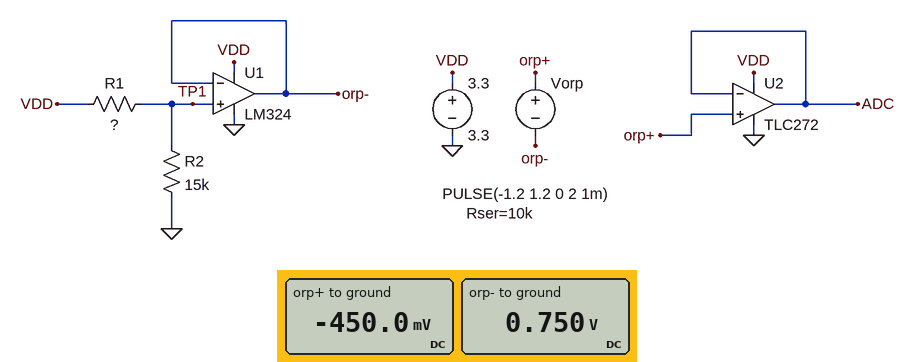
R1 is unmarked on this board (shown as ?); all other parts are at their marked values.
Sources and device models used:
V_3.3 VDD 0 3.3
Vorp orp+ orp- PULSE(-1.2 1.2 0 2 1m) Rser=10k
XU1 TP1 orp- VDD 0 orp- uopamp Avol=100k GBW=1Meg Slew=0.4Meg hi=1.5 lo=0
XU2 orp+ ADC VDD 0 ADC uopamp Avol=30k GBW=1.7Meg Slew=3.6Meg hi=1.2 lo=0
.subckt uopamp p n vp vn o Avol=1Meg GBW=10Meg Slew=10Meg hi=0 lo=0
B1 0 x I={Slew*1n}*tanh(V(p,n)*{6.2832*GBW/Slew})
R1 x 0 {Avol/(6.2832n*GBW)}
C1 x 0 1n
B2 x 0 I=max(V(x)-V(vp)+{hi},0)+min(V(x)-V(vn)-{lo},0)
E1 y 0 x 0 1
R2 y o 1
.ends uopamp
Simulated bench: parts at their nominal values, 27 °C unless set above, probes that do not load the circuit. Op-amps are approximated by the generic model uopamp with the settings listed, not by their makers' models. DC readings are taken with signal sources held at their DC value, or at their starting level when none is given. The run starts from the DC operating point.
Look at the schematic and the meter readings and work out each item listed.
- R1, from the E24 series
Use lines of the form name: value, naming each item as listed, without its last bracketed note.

R1, from the E24 series: 51 kΩ
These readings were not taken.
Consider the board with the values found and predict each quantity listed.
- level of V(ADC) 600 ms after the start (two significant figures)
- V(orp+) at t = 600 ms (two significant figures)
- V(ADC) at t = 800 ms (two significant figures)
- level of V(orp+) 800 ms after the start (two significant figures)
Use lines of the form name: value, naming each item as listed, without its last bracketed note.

level of V(ADC) 600 ms after the start: 270 mV
V(orp+) at t = 600 ms: 270 mV
V(ADC) at t = 800 ms: 510 mV
level of V(orp+) 800 ms after the start: 510 mV
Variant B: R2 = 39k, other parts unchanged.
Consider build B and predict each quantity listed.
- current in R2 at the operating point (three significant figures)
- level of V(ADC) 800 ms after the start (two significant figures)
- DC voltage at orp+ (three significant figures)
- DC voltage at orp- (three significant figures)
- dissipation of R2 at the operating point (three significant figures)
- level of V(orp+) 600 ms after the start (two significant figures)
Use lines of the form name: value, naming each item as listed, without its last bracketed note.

current in R2 at the operating point: 36.7 µA
level of V(ADC) 800 ms after the start: 1.2 V
DC voltage at orp+: 230 mV
DC voltage at orp-: 1.43 V
dissipation of R2 at the operating point: 52.4 µW
level of V(orp+) 600 ms after the start: 950 mV
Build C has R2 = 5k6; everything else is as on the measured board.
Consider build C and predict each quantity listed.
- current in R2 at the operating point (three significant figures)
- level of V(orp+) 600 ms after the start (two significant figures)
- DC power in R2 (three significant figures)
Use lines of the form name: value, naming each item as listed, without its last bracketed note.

current in R2 at the operating point: 58.3 µA
level of V(orp+) 600 ms after the start: -150 mV
DC power in R2: 19.0 µW
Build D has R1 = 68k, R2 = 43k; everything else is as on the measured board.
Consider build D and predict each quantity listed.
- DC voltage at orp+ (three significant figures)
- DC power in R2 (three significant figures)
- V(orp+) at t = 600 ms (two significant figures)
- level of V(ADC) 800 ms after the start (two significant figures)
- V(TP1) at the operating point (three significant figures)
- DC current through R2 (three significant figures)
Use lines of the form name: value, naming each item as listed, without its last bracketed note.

DC voltage at orp+: 78.4 mV
DC power in R2: 38.0 µW
V(orp+) at t = 600 ms: 800 mV
level of V(ADC) 800 ms after the start: 1.0 V
V(TP1) at the operating point: 1.28 V
DC current through R2: 29.7 µA
